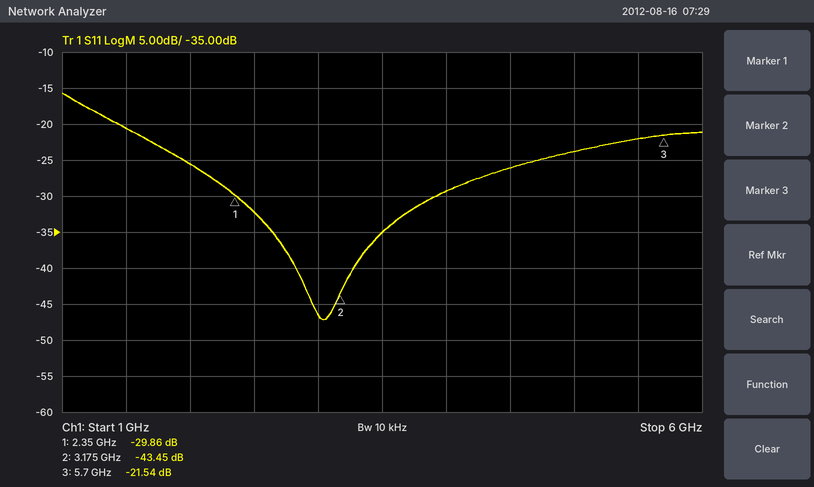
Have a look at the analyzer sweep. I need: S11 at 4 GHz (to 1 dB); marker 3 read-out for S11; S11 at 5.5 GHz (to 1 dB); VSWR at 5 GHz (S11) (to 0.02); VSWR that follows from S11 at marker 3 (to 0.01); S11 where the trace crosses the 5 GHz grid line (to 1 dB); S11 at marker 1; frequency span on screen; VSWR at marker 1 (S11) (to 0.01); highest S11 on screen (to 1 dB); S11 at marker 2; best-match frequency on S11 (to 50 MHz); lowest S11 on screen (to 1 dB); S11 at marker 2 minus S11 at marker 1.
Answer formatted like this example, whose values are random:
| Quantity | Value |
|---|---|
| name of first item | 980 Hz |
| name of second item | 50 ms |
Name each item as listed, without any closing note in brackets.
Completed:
| Quantity | Value |
|---|---|
| S11 at 4 GHz | -29 dB |
| marker 3 read-out for S11 | -21.54 dB |
| S11 at 5.5 GHz | -22 dB |
| VSWR at 5 GHz (S11) | 1.14 |
| VSWR that follows from S11 at marker 3 | 1.18 |
| S11 where the trace crosses the 5 GHz grid line | -24 dB |
| S11 at marker 1 | -29.86 dB |
| frequency span on screen | 5 GHz |
| VSWR at marker 1 (S11) | 1.07 |
| highest S11 on screen | -16 dB |
| S11 at marker 2 | -43.45 dB |
| best-match frequency on S11 | 3.05 GHz |
| lowest S11 on screen | -47 dB |
| S11 at marker 2 minus S11 at marker 1 | -13.59 dB |
